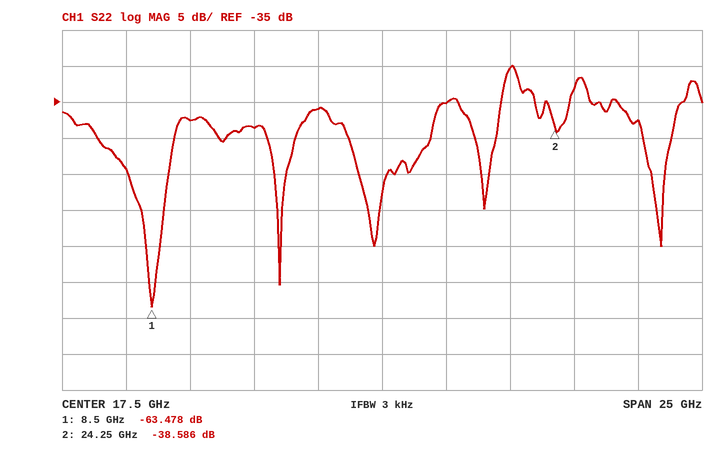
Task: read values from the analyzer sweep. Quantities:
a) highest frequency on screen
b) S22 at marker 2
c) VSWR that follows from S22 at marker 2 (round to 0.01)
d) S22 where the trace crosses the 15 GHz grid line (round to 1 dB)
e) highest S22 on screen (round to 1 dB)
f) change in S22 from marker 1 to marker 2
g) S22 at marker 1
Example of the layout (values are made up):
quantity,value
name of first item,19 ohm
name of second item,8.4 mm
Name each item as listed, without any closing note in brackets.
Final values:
quantity,value
highest frequency on screen,30 GHz
S22 at marker 2,-38.586 dB
VSWR that follows from S22 at marker 2,1.02
S22 where the trace crosses the 15 GHz grid line,-36 dB
highest S22 on screen,-30 dB
change in S22 from marker 1 to marker 2,24.892 dB
S22 at marker 1,-63.478 dB
